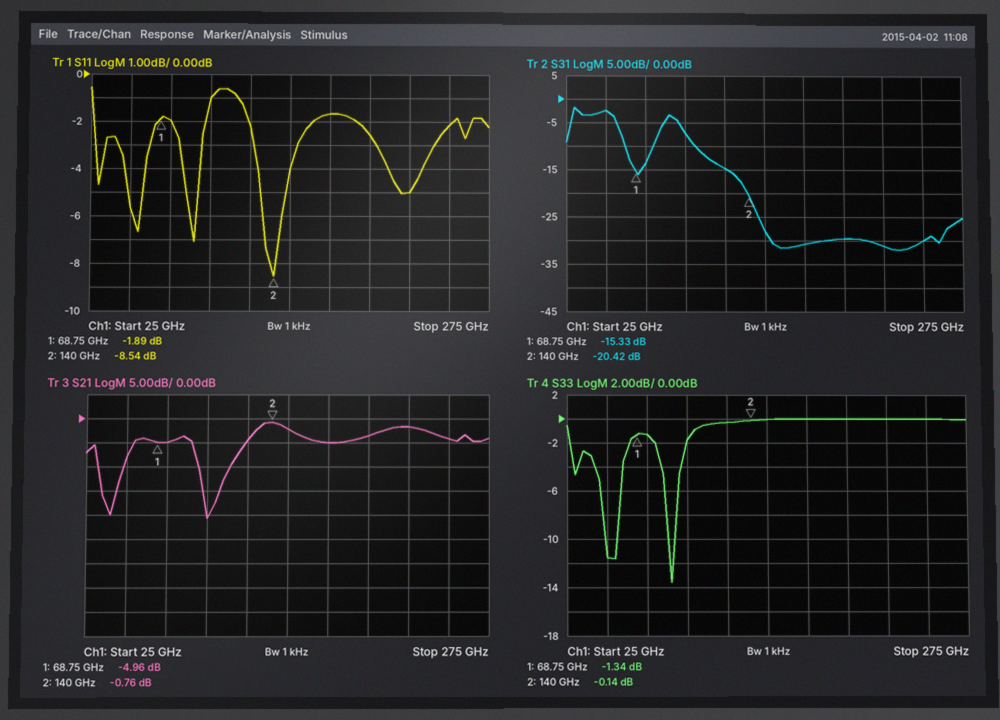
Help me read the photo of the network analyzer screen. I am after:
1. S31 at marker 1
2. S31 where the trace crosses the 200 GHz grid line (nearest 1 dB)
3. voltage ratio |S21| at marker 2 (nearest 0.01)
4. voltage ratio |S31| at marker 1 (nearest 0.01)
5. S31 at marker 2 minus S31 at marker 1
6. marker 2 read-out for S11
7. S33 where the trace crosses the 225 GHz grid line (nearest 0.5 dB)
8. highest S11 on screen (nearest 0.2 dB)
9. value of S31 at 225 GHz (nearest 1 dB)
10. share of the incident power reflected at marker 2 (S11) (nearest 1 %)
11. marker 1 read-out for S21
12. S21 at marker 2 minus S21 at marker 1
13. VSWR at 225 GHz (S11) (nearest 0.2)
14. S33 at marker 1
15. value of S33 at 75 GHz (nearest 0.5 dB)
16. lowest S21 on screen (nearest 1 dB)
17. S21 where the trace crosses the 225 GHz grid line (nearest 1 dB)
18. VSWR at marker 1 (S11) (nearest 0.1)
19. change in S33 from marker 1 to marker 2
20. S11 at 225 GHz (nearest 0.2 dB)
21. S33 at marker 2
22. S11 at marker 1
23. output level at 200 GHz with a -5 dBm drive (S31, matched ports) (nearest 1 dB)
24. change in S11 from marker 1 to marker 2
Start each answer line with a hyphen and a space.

- -15.33 dB
- -30 dB
- 0.92
- 0.17
- -5.09 dB
- -8.54 dB
- 0.0 dB
- -0.6 dB
- -31 dB
- 14 %
- -4.96 dB
- 4.20 dB
- 3.6
- -1.34 dB
- -1.5 dB
- -21 dB
- -2 dB
- 9.2
- 1.20 dB
- -5.0 dB
- -0.14 dB
- -1.89 dB
- -35 dBm
- -6.65 dB
